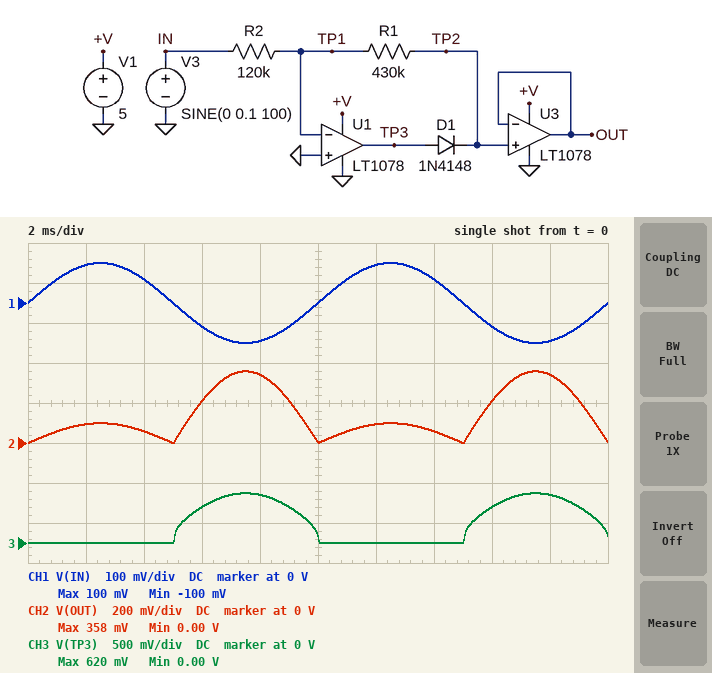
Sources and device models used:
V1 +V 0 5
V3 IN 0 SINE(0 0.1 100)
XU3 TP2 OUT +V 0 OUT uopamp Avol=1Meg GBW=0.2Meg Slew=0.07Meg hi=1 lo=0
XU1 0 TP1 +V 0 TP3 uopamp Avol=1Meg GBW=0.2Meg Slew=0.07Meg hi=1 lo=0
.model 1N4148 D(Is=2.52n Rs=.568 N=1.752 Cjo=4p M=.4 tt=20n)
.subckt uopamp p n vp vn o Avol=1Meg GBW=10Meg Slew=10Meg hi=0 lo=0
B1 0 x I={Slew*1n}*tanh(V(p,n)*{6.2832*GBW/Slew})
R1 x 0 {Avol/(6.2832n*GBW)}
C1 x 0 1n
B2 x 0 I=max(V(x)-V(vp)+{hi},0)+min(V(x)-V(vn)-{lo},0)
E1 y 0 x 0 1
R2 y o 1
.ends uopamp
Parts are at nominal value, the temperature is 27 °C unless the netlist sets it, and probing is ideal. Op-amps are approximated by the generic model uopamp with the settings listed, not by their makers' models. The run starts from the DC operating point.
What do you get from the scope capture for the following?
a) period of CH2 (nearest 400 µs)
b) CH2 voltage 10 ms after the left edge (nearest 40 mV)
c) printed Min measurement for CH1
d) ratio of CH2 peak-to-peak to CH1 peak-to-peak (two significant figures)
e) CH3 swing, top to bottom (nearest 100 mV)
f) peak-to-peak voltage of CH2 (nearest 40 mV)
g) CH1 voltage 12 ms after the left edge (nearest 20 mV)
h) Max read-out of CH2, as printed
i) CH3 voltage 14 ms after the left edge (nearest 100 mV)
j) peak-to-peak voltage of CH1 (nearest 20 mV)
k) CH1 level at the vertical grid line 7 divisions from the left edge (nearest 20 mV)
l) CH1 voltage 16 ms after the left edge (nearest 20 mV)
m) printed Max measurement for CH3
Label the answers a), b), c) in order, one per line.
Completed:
a) 10.0 ms
b) 0 V
c) -100 mV
d) 1.8
e) 600 mV
f) 360 mV
g) 100 mV
h) 358 mV
i) 0 V
j) 200 mV
k) 60 mV
l) -60 mV
m) 620 mV
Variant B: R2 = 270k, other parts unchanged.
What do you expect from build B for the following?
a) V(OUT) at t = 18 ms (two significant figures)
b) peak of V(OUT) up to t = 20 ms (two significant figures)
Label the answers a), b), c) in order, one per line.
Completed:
a) 150 mV
b) 160 mV
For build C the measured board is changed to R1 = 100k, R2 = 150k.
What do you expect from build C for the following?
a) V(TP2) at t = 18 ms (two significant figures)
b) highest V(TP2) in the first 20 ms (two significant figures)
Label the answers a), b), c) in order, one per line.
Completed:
a) 63 mV
b) 99 mV
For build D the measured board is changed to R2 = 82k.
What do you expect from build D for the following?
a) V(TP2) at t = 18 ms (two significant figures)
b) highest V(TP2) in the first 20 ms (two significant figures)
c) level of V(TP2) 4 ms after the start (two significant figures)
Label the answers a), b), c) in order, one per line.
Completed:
a) 500 mV
b) 520 mV
c) 58 mV
